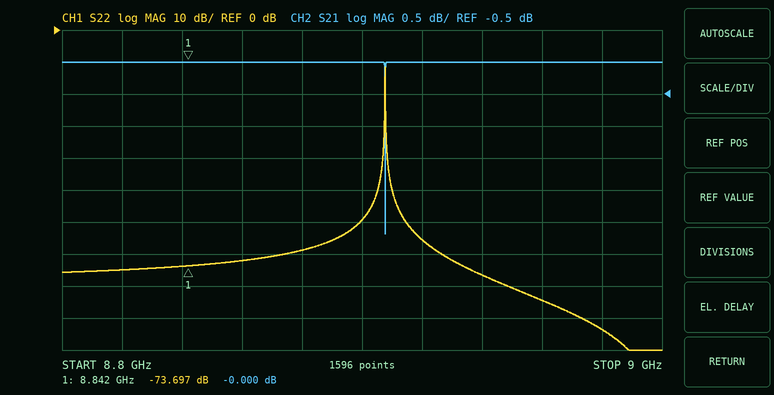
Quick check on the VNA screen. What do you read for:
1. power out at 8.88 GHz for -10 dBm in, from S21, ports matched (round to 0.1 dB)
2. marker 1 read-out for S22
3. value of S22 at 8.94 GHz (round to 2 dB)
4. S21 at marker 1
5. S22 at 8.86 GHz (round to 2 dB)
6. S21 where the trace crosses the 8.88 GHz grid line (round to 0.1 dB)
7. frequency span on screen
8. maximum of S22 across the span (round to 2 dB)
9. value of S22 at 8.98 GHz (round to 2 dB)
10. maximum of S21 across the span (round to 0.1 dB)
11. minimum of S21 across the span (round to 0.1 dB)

-10.0 dBm
-73.697 dB
-76 dB
-0.000 dB
-72 dB
0.0 dB
200 MHz
-12 dB
-94 dB
0.0 dB
-2.7 dB
